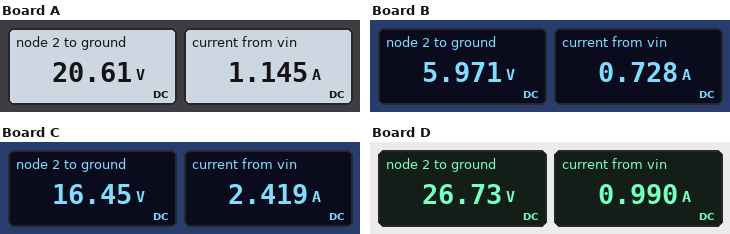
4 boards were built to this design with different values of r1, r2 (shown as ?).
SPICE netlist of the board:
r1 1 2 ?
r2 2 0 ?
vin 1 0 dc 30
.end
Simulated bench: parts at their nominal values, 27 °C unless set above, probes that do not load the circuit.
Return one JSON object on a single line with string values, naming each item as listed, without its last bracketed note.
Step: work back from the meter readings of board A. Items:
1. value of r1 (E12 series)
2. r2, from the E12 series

{"value of r1": "8.2 Ω", "r2, from the E12 series": "18 Ω"}
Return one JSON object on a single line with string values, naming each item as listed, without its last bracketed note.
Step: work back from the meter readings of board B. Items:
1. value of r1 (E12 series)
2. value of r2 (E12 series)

{"value of r1": "33 Ω", "value of r2": "8.2 Ω"}
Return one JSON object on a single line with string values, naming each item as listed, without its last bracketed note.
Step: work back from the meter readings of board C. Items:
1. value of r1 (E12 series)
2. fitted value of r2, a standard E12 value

{"value of r1": "5.6 Ω", "fitted value of r2, a standard E12 value": "6.8 Ω"}
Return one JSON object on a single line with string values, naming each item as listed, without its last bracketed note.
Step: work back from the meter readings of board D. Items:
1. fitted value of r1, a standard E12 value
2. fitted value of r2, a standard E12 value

{"fitted value of r1, a standard E12 value": "3.3 Ω", "fitted value of r2, a standard E12 value": "27 Ω"}
